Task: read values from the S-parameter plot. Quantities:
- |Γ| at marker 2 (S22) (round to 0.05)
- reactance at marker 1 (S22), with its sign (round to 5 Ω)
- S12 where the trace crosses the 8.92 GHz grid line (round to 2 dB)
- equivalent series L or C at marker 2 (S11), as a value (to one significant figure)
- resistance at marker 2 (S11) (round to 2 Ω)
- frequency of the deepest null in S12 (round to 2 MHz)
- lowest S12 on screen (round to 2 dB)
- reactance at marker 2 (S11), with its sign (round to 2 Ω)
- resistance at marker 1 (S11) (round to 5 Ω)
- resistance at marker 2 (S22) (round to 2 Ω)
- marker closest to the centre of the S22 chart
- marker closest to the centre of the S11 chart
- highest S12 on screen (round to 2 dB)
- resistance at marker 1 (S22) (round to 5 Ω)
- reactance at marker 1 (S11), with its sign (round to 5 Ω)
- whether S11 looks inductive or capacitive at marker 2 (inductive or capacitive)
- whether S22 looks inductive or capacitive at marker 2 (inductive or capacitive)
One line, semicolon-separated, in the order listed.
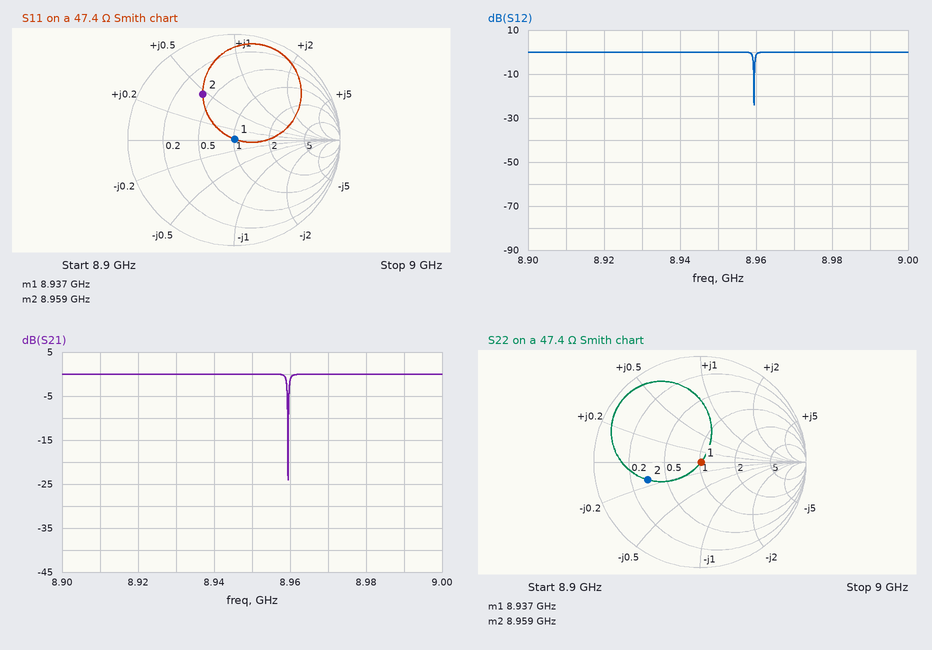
0.50; 0 Ω; 0 dB; 400 pH; 18 Ω; 8.960 GHz; -24 dB; +22 Ω; 50 Ω; 16 Ω; marker 1; marker 1; 0 dB; 50 Ω; 0 Ω; inductive; capacitive
